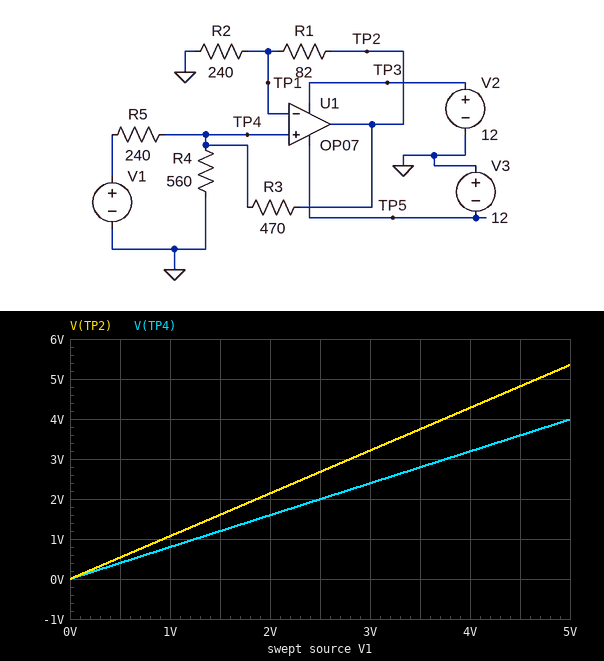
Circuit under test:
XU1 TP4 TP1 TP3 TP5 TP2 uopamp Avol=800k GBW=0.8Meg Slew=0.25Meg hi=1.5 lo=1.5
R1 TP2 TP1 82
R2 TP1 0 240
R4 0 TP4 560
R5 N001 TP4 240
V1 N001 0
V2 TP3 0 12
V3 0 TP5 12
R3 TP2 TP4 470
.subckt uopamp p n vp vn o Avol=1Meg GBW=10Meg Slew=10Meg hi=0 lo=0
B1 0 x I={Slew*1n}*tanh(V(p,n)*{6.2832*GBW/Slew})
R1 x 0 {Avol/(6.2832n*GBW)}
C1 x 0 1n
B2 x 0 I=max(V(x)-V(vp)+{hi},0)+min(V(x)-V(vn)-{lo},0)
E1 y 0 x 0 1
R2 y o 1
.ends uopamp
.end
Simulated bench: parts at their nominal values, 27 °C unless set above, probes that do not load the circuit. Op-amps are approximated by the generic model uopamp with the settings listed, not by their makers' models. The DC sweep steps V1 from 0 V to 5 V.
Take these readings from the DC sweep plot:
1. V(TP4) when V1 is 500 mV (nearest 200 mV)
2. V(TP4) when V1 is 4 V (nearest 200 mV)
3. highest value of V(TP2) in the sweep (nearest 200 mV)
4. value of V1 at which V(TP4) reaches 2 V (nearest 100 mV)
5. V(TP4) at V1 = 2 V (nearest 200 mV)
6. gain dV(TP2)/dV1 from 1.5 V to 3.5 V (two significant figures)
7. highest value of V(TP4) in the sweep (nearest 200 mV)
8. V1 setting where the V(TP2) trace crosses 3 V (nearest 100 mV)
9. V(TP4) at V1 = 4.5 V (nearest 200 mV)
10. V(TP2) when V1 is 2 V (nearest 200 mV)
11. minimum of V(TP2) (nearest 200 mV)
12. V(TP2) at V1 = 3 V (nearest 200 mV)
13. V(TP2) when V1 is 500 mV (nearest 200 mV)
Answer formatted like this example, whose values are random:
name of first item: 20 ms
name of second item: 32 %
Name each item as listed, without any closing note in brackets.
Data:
V(TP4) when V1 is 500 mV: 400 mV
V(TP4) when V1 is 4 V: 3.2 V
highest value of V(TP2) in the sweep: 5.4 V
value of V1 at which V(TP4) reaches 2 V: 2.5 V
V(TP4) at V1 = 2 V: 1.6 V
gain dV(TP2)/dV1 from 1.5 V to 3.5 V: 1.1 V/V
highest value of V(TP4) in the sweep: 4.0 V
V1 setting where the V(TP2) trace crosses 3 V: 2.8 V
V(TP4) at V1 = 4.5 V: 3.6 V
V(TP2) when V1 is 2 V: 2.2 V
minimum of V(TP2): 0 V
V(TP2) at V1 = 3 V: 3.2 V
V(TP2) when V1 is 500 mV: 600 mV
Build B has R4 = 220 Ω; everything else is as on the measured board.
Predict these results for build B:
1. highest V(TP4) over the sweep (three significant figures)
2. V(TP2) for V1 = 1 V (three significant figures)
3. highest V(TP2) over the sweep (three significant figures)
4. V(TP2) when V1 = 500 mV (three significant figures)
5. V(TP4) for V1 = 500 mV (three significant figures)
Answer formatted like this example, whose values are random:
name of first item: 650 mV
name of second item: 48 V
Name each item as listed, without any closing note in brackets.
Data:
highest V(TP4) over the sweep: 2.61 V
V(TP2) for V1 = 1 V: 700 mV
highest V(TP2) over the sweep: 3.50 V
V(TP2) when V1 = 500 mV: 350 mV
V(TP4) for V1 = 500 mV: 261 mV
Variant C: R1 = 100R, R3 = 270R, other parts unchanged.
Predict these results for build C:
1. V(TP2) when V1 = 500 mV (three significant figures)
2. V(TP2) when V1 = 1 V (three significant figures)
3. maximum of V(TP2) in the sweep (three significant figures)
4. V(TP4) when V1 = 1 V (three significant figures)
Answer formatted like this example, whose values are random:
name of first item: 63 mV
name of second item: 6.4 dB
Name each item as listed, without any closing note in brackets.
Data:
V(TP2) when V1 = 500 mV: 669 mV
V(TP2) when V1 = 1 V: 1.34 V
maximum of V(TP2) in the sweep: 6.69 V
V(TP4) when V1 = 1 V: 945 mV
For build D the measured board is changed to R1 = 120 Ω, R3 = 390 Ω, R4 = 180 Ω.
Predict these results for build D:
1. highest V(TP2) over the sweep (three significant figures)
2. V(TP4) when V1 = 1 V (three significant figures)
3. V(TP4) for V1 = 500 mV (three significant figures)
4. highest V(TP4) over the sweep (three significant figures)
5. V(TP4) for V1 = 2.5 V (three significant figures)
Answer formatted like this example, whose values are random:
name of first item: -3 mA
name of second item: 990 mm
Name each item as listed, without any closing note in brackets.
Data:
highest V(TP2) over the sweep: 3.70 V
V(TP4) when V1 = 1 V: 494 mV
V(TP4) for V1 = 500 mV: 247 mV
highest V(TP4) over the sweep: 2.47 V
V(TP4) for V1 = 2.5 V: 1.23 V
